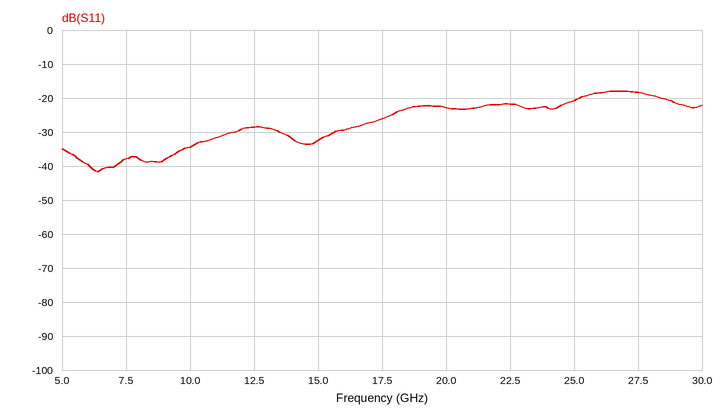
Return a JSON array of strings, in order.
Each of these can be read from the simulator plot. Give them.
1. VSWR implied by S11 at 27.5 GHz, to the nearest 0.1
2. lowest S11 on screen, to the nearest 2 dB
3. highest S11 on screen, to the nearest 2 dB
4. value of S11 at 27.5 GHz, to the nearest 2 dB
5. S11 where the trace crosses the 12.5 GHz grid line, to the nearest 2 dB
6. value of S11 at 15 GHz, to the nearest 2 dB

["1.3", "-42 dB", "-18 dB", "-18 dB", "-28 dB", "-32 dB"]
